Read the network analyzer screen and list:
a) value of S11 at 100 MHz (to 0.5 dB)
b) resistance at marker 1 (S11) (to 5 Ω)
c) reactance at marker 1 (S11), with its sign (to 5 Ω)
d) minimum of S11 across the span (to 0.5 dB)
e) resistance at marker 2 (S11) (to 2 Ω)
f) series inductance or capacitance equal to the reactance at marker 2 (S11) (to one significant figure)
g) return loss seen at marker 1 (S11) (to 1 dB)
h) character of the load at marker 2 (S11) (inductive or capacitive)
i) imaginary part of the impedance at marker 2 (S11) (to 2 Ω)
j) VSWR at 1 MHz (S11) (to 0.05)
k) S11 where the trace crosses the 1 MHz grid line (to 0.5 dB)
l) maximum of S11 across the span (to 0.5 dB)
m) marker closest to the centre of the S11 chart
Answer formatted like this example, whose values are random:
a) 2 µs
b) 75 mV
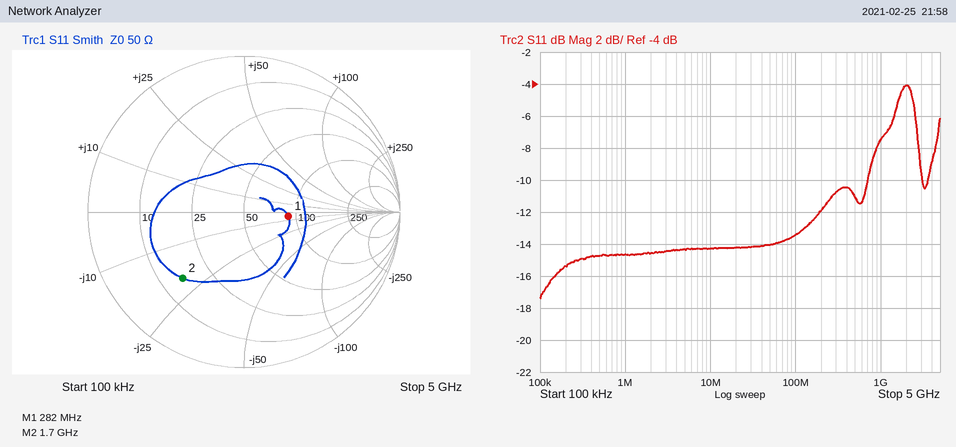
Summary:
a) -13.5 dB
b) 90 Ω
c) -5 Ω
d) -17.5 dB
e) 16 Ω
f) 5 pF
g) 11 dB
h) capacitive
i) -20 Ω
j) 1.45
k) -14.5 dB
l) -4.0 dB
m) marker 1
